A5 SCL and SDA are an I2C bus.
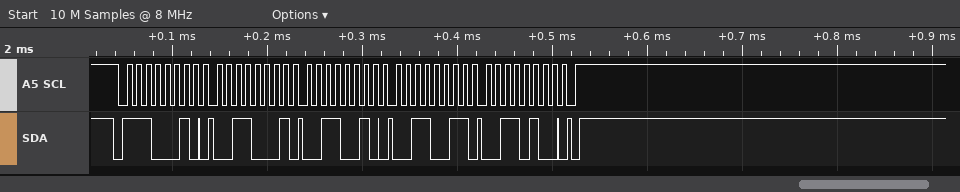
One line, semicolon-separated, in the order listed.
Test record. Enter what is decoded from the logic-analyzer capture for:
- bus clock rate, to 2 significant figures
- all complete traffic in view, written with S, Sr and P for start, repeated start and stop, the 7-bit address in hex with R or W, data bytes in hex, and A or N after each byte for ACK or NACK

100 kHz; S 71W A 31 A 32 A 33 A 34 A P
